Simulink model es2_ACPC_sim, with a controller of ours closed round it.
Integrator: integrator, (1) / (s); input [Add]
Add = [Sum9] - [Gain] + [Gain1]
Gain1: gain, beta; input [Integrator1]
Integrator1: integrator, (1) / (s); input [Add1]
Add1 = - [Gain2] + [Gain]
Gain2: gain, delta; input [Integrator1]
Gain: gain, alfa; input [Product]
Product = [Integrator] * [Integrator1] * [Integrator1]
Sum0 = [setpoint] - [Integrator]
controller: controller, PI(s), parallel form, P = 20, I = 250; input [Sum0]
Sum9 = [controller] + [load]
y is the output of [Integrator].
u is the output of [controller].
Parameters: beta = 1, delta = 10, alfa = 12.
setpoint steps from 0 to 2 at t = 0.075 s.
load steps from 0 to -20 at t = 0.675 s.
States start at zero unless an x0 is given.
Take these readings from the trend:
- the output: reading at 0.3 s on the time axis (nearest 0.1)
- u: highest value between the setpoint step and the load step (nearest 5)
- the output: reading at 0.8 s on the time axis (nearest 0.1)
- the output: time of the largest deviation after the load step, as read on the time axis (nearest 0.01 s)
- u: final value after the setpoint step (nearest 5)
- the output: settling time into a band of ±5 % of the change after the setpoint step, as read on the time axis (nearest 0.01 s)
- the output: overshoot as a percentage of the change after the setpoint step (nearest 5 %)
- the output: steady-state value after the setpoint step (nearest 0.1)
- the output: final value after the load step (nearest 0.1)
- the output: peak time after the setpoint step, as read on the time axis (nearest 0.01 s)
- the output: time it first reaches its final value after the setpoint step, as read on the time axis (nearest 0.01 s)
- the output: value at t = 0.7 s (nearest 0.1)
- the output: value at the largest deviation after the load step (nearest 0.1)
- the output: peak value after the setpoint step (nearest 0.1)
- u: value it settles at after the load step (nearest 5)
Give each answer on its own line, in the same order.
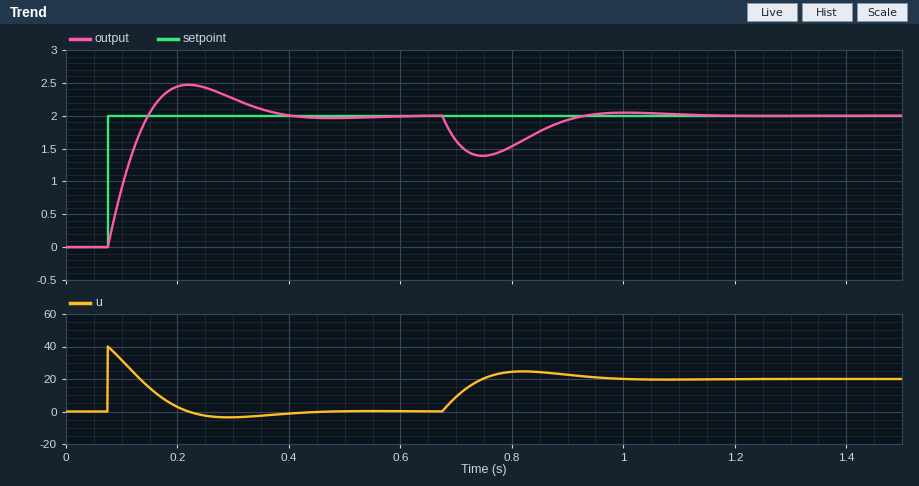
2.3
40
1.5
0.75 s
0
0.35 s
25 %
2.0
2.0
0.22 s
0.15 s
1.6
1.4
2.5
20
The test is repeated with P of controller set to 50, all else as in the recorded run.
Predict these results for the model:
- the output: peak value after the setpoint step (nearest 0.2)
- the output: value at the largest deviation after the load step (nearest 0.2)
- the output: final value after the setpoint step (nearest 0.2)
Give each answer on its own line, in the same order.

2.2
1.6
2.0
